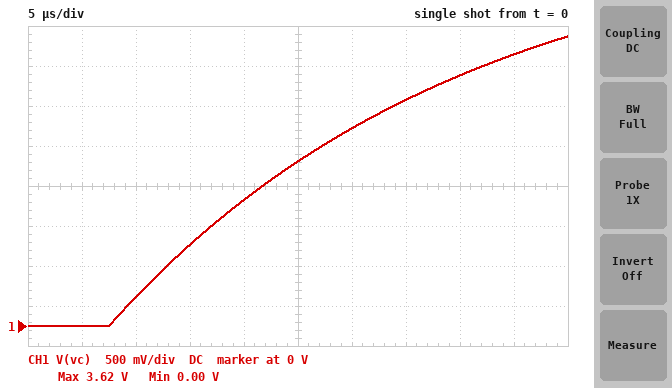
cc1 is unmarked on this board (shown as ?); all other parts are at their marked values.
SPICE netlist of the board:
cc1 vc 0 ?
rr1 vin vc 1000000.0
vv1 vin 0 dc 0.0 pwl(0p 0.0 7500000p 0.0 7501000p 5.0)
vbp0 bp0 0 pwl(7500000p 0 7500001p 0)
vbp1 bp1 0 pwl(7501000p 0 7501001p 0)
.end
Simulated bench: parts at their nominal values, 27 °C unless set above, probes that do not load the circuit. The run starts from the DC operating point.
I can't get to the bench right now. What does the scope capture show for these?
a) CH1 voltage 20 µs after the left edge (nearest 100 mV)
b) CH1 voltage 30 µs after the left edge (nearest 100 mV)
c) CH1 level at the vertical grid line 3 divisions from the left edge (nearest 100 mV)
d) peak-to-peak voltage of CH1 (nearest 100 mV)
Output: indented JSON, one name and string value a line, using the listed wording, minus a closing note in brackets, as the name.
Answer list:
{
  "CH1 voltage 20 µs after the left edge": "1.6 V",
  "CH1 voltage 30 µs after the left edge": "2.5 V",
  "CH1 level at the vertical grid line 3 divisions from the left edge": "1.0 V",
  "peak-to-peak voltage of CH1": "3.6 V"
}
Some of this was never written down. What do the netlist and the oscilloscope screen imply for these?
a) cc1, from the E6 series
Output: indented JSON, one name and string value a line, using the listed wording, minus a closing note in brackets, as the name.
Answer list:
{
  "cc1, from the E6 series": "33 pF"
}
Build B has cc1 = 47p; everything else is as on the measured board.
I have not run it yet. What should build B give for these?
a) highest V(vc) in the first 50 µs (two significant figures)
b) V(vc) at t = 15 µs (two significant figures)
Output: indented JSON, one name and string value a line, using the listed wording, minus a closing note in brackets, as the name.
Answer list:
{
  "highest V(vc) in the first 50 µs": "3.0 V",
  "V(vc) at t = 15 µs": "740 mV"
}
